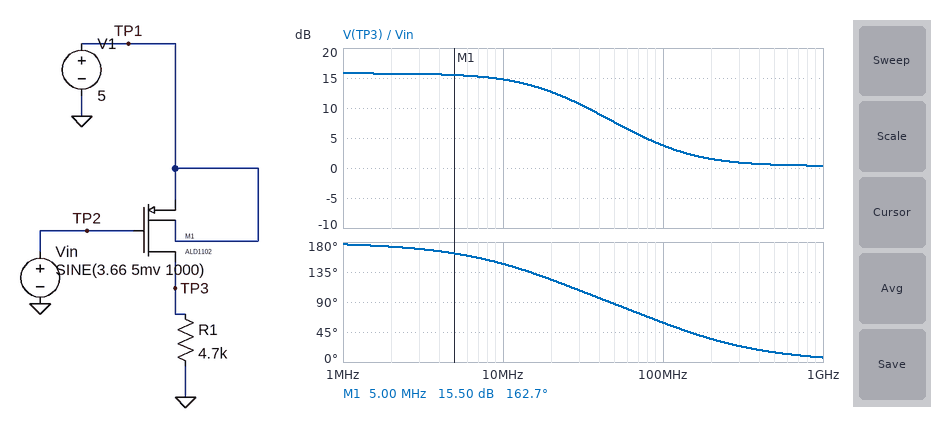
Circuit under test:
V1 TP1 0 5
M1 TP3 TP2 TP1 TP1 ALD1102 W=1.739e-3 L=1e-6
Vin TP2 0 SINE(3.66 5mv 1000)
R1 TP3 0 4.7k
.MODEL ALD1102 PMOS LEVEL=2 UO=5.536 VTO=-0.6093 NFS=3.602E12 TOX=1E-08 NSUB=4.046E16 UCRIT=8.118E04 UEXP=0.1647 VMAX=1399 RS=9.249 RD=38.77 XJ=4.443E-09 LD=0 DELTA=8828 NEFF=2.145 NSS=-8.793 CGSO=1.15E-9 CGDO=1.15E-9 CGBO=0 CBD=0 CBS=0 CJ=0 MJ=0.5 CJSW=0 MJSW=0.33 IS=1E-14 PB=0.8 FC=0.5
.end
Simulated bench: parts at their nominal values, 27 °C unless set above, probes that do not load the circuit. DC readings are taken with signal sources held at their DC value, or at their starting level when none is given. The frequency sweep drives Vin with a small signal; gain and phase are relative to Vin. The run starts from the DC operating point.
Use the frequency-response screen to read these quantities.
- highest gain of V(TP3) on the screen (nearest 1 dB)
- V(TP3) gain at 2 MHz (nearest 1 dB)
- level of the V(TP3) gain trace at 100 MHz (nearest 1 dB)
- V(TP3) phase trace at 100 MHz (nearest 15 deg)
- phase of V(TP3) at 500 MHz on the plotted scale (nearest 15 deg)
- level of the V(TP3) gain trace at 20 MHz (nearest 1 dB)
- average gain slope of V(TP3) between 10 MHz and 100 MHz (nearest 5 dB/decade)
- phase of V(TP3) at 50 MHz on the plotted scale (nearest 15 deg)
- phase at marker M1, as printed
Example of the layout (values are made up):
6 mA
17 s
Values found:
16 dB
16 dB
4 dB
60 deg
15 deg
13 dB
-10 dB/decade
90 deg
162.7 deg
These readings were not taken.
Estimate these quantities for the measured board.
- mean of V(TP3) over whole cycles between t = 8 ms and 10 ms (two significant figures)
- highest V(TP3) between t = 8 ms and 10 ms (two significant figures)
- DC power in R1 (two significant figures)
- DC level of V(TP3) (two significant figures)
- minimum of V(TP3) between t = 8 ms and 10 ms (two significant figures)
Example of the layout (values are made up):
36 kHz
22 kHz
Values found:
2.6 V
2.6 V
1.4 mW
2.6 V
2.5 V
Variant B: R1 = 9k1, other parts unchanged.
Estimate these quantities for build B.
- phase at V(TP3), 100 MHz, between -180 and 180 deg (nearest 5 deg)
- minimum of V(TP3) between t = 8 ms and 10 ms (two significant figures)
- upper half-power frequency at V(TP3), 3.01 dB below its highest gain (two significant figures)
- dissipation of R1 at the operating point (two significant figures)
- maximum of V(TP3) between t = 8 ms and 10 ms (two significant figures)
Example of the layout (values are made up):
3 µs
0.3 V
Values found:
50 deg
4.3 V
14 MHz
2.1 mW
4.4 V
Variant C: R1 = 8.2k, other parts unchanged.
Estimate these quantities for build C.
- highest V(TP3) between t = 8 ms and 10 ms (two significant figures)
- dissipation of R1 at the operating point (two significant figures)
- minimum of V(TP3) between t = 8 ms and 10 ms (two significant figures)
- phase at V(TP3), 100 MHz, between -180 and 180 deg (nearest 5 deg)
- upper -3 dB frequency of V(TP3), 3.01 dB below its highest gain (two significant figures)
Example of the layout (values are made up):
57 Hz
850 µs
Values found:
4.1 V
2.0 mW
4.0 V
55 deg
14 MHz
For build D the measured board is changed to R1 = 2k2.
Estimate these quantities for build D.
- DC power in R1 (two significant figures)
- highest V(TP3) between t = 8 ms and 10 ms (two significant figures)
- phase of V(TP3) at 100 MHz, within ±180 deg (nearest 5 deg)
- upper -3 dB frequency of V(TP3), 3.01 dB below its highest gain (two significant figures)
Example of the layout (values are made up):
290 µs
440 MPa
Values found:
740 µW
1.3 V
70 deg
42 MHz
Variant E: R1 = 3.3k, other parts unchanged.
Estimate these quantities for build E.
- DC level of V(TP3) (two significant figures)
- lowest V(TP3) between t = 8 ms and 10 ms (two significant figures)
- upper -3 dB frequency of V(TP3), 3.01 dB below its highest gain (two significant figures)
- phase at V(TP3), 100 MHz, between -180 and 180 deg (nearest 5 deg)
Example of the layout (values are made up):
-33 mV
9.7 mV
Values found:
1.9 V
1.8 V
27 MHz
65 deg
